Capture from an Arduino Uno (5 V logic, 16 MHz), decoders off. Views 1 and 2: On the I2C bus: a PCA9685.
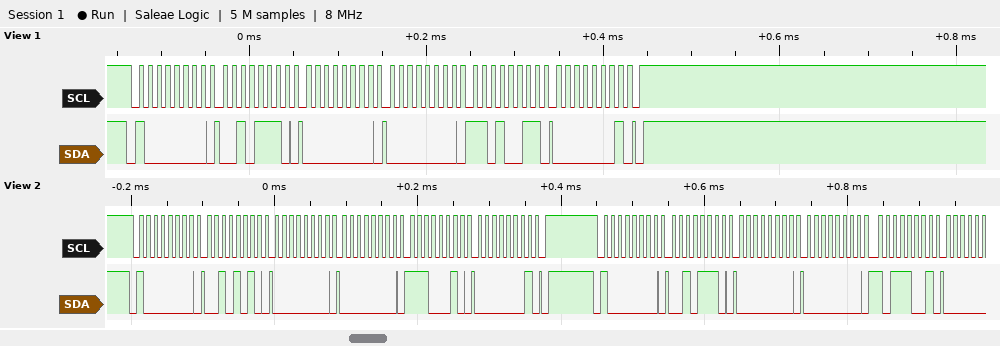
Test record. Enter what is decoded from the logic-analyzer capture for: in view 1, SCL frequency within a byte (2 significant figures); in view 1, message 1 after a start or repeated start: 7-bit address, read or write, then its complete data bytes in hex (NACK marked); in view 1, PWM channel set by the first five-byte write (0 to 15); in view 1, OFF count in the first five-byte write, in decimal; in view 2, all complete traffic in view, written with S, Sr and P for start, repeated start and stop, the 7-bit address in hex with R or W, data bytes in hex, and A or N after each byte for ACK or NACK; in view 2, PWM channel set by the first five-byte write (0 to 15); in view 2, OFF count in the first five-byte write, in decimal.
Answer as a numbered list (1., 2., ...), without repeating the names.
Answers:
1. 100 kHz
2. 0x40 write: 2E 00 00 D3 01
3. 10
4. 467
5. S 40W A 2A A 00 A 00 A E2 A 01 A P S 40W A 2E A 00 A 00 A B9 A
6. 9
7. 482
